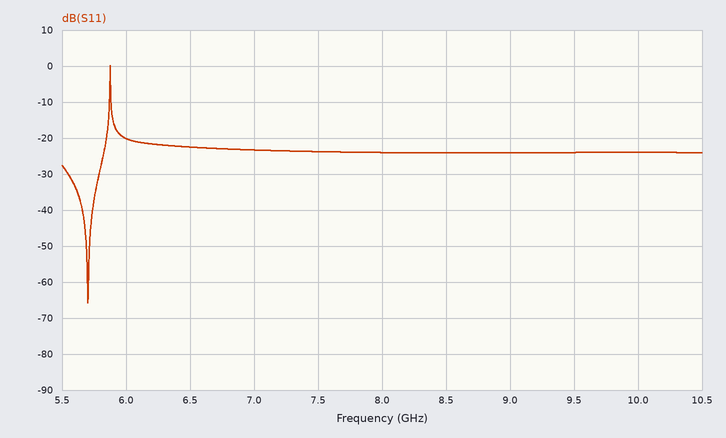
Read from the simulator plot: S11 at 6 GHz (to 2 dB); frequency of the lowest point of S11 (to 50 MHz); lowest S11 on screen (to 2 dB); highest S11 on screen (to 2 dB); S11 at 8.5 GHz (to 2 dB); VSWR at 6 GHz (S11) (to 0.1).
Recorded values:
-20 dB
5.70 GHz
-66 dB
0 dB
-24 dB
1.2
